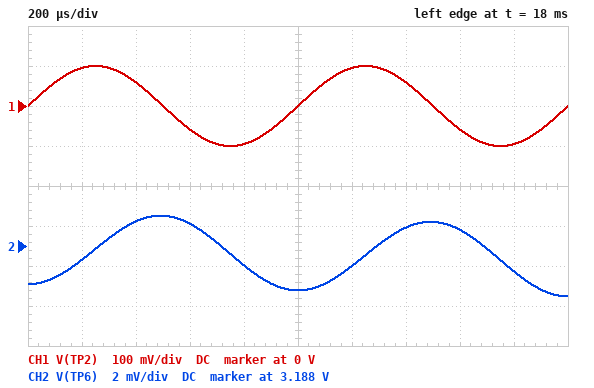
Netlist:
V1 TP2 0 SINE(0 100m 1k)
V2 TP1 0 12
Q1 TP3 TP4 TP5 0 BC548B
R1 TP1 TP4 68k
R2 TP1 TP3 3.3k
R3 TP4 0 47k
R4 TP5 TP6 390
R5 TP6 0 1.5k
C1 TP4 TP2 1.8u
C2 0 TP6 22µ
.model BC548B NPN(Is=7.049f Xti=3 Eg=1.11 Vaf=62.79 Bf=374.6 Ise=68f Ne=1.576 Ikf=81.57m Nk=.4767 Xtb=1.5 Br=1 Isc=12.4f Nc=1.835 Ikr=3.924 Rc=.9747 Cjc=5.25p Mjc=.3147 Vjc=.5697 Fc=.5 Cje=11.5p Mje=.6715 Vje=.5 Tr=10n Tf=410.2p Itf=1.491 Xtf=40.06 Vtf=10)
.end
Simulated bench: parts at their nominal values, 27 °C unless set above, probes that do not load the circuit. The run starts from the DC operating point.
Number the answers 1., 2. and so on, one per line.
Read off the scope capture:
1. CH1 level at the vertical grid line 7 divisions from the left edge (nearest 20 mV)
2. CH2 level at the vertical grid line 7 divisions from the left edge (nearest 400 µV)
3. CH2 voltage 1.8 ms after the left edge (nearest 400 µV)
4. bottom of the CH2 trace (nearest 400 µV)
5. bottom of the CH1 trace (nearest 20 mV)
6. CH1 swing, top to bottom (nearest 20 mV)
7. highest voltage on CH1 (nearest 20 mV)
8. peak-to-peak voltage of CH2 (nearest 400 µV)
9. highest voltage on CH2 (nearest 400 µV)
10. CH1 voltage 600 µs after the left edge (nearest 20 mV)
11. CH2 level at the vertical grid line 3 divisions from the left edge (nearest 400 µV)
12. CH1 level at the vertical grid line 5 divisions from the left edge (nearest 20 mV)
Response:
1. 60 mV
2. 3.1888 V
3. 3.1868 V
4. 3.1856 V
5. -100 mV
6. 200 mV
7. 100 mV
8. 4.0 mV
9. 3.1896 V
10. -60 mV
11. 3.1892 V
12. 0 V
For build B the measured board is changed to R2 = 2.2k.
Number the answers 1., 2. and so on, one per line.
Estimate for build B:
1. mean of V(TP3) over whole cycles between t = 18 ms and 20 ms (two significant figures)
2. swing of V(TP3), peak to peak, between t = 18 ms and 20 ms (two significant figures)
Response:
1. 7.3 V
2. 1.1 V
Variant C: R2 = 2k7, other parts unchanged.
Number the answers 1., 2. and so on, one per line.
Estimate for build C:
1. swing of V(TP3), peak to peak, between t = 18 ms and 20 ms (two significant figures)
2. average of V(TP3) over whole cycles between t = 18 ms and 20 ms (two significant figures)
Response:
1. 1.3 V
2. 6.3 V
